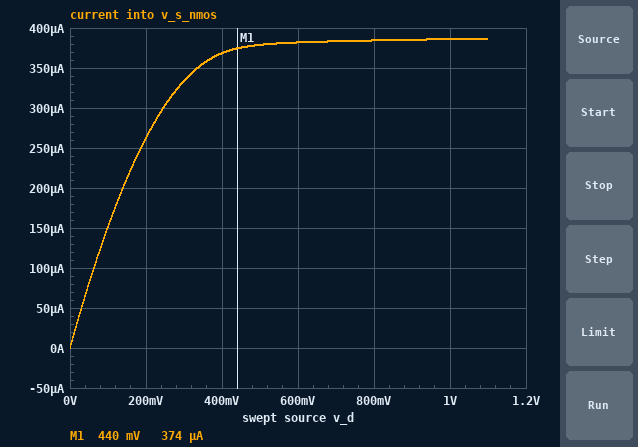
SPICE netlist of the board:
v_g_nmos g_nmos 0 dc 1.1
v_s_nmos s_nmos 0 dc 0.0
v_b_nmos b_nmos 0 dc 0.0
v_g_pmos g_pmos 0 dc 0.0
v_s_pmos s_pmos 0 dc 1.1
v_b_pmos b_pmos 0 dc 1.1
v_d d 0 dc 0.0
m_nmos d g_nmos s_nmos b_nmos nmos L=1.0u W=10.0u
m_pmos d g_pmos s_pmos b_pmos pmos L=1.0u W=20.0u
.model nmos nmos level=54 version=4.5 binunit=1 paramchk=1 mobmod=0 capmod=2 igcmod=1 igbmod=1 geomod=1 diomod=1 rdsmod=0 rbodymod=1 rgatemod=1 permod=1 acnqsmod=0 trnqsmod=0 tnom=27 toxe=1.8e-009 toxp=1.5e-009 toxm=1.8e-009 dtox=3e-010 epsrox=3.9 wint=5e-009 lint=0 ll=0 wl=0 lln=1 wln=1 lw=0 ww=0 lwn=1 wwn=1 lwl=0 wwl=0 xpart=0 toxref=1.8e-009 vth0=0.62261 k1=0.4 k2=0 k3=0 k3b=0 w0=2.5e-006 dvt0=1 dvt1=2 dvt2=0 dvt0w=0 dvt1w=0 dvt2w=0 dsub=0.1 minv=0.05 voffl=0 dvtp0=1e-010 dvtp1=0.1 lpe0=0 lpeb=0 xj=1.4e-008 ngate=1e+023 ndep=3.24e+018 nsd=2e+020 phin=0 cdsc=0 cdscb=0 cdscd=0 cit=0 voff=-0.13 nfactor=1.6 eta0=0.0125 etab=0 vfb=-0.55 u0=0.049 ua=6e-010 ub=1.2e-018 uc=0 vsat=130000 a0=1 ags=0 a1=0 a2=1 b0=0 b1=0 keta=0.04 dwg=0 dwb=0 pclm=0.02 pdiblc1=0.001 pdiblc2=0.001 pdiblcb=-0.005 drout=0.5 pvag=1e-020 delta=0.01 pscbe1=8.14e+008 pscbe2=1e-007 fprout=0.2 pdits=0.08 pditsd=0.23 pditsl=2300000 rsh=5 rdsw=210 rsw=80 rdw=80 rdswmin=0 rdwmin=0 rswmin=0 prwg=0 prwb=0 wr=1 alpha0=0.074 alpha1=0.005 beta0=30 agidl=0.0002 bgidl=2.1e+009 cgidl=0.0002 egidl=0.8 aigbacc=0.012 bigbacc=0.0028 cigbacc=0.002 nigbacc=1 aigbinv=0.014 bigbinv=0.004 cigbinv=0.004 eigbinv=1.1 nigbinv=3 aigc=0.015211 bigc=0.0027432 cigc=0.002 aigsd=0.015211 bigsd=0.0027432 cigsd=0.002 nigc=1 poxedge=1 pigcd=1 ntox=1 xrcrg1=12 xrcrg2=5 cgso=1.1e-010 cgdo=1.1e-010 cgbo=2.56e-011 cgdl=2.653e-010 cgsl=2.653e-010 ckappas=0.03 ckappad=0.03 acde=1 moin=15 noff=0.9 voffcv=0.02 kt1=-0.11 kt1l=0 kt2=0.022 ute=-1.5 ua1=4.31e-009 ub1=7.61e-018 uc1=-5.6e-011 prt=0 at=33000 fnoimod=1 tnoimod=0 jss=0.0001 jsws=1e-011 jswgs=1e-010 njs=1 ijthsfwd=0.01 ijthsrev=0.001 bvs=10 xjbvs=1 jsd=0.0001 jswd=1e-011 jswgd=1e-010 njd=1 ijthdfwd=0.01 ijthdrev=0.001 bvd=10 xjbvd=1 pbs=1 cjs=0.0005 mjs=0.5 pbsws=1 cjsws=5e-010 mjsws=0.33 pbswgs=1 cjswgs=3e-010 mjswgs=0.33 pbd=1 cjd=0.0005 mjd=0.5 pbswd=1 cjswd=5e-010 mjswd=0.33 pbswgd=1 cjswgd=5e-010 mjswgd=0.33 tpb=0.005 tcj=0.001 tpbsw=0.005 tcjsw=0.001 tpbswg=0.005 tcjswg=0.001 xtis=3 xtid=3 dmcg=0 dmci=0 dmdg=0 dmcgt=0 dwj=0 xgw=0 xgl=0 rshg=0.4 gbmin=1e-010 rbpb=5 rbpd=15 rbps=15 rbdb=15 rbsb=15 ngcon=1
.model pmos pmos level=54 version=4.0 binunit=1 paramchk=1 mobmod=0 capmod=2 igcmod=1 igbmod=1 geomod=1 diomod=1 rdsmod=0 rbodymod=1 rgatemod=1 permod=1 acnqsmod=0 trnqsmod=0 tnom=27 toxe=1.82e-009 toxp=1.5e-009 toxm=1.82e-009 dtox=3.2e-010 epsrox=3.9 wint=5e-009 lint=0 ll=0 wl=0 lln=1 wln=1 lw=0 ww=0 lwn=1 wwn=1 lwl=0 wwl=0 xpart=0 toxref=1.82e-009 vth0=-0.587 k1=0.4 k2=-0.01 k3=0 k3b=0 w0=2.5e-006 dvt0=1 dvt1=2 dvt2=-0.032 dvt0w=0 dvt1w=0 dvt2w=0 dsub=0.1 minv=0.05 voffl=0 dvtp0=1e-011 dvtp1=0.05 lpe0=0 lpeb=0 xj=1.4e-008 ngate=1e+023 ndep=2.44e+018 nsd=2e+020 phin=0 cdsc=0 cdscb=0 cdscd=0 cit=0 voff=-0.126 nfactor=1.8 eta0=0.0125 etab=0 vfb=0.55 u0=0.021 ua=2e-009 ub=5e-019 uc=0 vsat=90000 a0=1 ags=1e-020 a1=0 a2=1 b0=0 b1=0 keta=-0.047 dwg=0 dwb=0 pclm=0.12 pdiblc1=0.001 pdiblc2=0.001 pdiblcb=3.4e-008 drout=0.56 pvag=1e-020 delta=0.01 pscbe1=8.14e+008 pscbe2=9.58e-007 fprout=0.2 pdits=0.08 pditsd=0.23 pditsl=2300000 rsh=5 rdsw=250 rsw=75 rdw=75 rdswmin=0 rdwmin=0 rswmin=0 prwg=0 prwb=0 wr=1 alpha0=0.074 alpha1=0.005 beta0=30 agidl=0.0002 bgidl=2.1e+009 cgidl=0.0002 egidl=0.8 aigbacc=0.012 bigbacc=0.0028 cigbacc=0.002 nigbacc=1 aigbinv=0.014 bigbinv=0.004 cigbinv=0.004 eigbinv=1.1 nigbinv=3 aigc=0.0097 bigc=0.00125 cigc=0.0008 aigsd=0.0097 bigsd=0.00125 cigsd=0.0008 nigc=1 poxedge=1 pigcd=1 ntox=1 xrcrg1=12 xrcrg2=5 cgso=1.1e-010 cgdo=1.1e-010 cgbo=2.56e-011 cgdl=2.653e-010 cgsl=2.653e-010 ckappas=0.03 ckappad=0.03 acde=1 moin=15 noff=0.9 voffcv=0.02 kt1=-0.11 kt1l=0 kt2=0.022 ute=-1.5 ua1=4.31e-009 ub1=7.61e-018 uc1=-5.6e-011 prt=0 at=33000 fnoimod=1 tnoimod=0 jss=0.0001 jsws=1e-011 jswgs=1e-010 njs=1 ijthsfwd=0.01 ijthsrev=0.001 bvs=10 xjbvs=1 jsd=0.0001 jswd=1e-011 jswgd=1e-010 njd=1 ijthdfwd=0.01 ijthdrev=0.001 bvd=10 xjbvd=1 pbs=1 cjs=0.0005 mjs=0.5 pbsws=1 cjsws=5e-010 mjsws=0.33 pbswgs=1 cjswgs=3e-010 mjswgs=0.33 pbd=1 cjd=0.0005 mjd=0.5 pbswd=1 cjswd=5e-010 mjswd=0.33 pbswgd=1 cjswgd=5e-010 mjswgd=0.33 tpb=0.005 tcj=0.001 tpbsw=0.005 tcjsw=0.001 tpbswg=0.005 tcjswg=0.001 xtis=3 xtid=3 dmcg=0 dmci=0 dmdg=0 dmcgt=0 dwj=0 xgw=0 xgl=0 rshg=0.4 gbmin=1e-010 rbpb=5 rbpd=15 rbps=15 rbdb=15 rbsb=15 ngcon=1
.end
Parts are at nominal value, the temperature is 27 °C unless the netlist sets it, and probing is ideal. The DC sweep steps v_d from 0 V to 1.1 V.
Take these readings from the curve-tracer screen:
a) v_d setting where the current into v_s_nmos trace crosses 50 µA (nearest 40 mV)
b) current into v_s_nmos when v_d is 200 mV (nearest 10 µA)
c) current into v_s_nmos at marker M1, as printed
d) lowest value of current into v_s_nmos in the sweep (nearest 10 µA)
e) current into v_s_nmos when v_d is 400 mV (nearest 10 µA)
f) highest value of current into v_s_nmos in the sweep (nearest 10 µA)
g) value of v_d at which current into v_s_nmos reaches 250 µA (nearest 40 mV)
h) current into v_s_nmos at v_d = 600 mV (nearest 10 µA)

40 mV
260 µA
374 µA
0 A
370 µA
390 µA
200 mV
380 µA
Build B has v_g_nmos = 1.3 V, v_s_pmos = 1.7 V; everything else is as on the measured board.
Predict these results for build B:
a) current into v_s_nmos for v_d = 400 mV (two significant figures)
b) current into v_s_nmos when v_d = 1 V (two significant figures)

570 µA
660 µA
